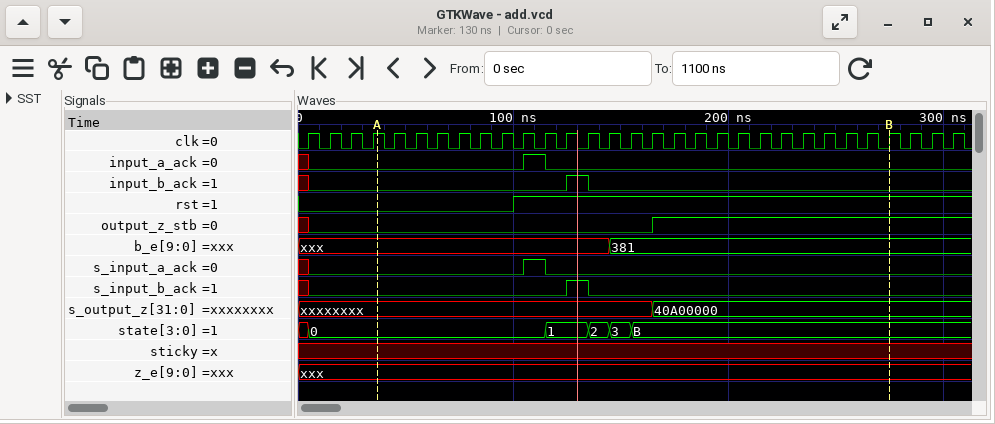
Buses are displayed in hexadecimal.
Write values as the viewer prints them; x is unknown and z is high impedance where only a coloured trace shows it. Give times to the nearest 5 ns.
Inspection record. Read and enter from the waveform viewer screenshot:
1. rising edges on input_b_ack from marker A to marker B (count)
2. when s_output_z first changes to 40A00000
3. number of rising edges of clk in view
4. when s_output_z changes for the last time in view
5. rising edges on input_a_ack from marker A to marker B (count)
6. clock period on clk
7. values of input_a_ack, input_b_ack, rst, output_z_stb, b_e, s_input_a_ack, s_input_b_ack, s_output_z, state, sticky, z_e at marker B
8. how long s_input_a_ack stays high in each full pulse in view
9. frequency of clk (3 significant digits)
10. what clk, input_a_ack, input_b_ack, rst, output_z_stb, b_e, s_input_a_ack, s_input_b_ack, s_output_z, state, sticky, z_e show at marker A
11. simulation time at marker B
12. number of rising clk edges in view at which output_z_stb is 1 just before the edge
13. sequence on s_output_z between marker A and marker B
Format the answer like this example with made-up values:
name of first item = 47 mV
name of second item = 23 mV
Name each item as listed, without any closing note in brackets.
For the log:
rising edges on input_b_ack from marker A to marker B = 1
when s_output_z first changes to 40A00000 = 165 ns
number of rising edges of clk in view = 31
when s_output_z changes for the last time in view = 165 ns
rising edges on input_a_ack from marker A to marker B = 1
clock period on clk = 10 ns
values of input_a_ack, input_b_ack, rst, output_z_stb, b_e, s_input_a_ack, s_input_b_ack, s_output_z, state, sticky, z_e at marker B = input_a_ack=0, input_b_ack=0, rst=1, output_z_stb=1, b_e=381, s_input_a_ack=0, s_input_b_ack=0, s_output_z=40A00000, state=B, sticky=x, z_e=xxx
how long s_input_a_ack stays high in each full pulse in view = 10 ns
frequency of clk = 100 MHz
what clk, input_a_ack, input_b_ack, rst, output_z_stb, b_e, s_input_a_ack, s_input_b_ack, s_output_z, state, sticky, z_e show at marker A = clk=1, input_a_ack=0, input_b_ack=0, rst=0, output_z_stb=0, b_e=xxx, s_input_a_ack=0, s_input_b_ack=0, s_output_z=xxxxxxxx, state=0, sticky=x, z_e=xxx
simulation time at marker B = 275 ns
number of rising clk edges in view at which output_z_stb is 1 just before the edge = 14
sequence on s_output_z between marker A and marker B = xxxxxxxx, 40A00000
